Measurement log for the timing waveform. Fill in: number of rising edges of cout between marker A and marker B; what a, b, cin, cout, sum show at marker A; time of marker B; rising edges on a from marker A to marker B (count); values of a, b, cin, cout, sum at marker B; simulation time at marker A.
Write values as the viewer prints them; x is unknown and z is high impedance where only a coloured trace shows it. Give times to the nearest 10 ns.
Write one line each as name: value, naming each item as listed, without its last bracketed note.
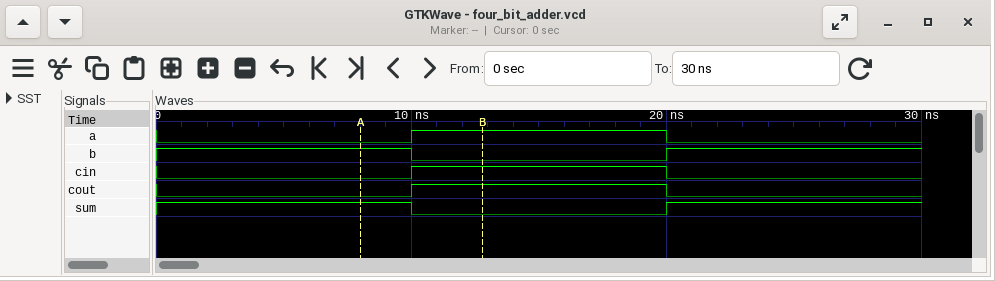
number of rising edges of cout between marker A and marker B: 1
what a, b, cin, cout, sum show at marker A: a=0, b=1, cin=0, cout=0, sum=1
time of marker B: 10 ns
rising edges on a from marker A to marker B: 1
values of a, b, cin, cout, sum at marker B: a=1, b=0, cin=1, cout=1, sum=0
simulation time at marker A: 10 ns
